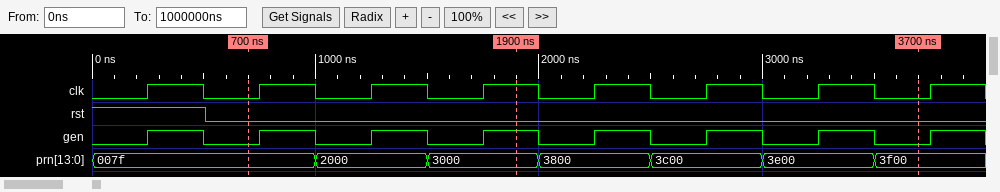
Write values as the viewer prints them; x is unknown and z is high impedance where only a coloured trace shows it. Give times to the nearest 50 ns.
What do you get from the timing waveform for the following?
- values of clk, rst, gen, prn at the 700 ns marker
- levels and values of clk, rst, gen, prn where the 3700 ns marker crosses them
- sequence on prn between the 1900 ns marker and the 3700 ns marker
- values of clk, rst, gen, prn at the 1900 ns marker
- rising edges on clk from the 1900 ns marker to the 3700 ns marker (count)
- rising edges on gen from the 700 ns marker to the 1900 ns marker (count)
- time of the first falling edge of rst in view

clk=0, rst=0, gen=0, prn=007f
clk=0, rst=0, gen=0, prn=3f00
3000, 3800, 3c00, 3e00, 3f00
clk=1, rst=0, gen=1, prn=3000
3
3
500 ns
